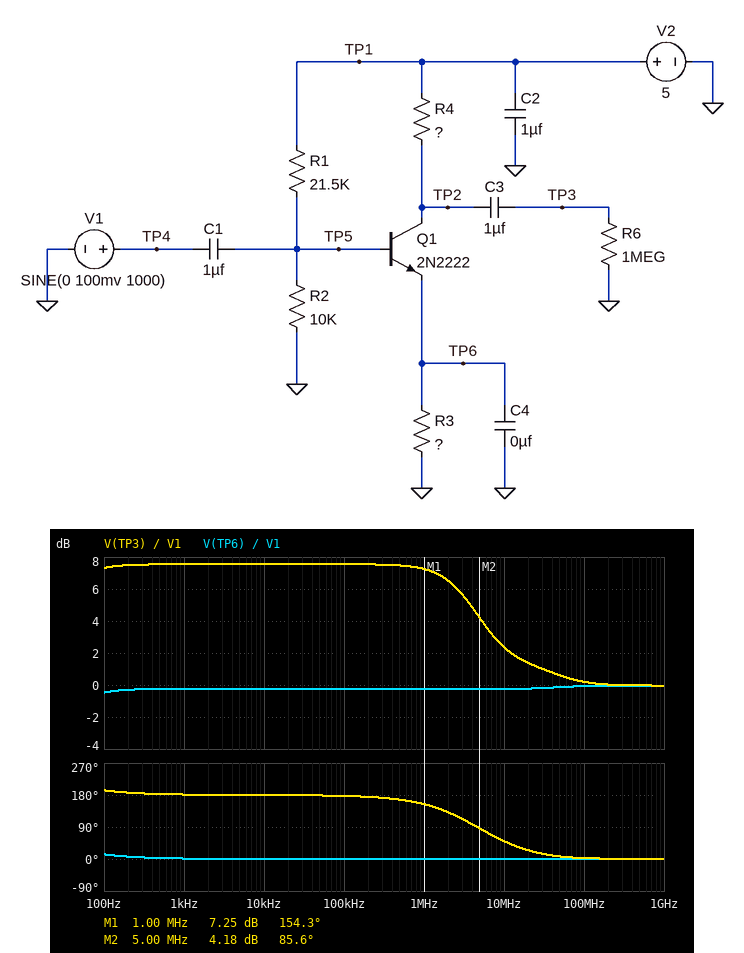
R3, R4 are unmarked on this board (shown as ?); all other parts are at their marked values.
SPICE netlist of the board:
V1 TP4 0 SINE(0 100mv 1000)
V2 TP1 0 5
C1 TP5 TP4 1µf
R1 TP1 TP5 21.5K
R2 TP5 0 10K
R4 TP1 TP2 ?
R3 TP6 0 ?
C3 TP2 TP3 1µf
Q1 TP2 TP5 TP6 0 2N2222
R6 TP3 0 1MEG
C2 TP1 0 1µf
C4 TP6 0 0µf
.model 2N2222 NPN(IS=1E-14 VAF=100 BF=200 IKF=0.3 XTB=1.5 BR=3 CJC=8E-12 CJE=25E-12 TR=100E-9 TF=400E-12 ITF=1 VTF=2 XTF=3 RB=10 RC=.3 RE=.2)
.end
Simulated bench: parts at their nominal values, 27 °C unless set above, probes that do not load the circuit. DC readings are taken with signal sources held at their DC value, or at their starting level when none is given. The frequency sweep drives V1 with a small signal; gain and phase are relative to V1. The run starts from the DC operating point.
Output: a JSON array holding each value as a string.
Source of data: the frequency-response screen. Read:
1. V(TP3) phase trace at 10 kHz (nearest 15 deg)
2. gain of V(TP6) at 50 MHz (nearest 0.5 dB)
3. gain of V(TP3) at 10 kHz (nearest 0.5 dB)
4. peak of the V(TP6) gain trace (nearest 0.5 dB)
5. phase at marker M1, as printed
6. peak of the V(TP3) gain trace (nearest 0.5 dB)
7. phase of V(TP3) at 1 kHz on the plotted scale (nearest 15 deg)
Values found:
["180 deg", "0 dB", "7.5 dB", "0 dB", "154.3 deg", "7.5 dB", "180 deg"]
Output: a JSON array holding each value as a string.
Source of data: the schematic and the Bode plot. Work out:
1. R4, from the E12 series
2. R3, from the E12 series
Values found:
["8.2 kΩ", "3.3 kΩ"]
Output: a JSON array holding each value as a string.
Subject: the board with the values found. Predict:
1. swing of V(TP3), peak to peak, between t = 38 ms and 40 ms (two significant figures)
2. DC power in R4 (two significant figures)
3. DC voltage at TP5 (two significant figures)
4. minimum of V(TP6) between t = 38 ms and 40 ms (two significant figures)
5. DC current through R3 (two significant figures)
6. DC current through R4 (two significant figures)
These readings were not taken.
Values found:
["480 mV", "680 µW", "1.6 V", "860 mV", "290 µA", "290 µA"]
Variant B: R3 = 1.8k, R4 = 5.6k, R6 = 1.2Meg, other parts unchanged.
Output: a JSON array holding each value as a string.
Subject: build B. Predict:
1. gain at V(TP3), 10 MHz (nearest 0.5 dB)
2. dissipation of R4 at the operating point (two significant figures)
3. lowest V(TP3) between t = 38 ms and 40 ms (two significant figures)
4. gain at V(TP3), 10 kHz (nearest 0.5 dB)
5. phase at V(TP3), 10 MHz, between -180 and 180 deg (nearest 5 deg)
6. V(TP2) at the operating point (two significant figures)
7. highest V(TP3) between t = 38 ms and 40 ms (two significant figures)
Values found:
["4.0 dB", "1.5 mW", "-300 mV", "9.5 dB", "70 deg", "2.1 V", "300 mV"]
